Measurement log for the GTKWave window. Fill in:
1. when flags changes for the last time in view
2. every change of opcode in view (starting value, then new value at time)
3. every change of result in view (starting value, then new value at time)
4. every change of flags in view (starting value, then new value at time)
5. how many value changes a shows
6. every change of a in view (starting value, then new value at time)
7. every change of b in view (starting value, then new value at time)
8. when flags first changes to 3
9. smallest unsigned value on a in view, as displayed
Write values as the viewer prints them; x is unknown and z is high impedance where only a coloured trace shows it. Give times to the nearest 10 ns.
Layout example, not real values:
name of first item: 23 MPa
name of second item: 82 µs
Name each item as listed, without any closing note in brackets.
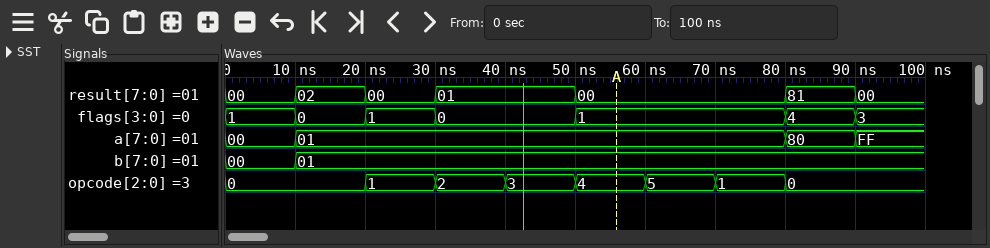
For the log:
when flags changes for the last time in view: 90 ns
every change of opcode in view: 0, 1 at 20 ns, 2 at 30 ns, 3 at 40 ns, 4 at 50 ns, 5 at 60 ns, 1 at 70 ns, 0 at 80 ns
every change of result in view: 00, 02 at 10 ns, 00 at 20 ns, 01 at 30 ns, 00 at 50 ns, 81 at 80 ns, 00 at 90 ns
every change of flags in view: 1, 0 at 10 ns, 1 at 20 ns, 0 at 30 ns, 1 at 50 ns, 4 at 80 ns, 3 at 90 ns
how many value changes a shows: 3
every change of a in view: 00, 01 at 10 ns, 80 at 80 ns, FF at 90 ns
every change of b in view: 00, 01 at 10 ns
when flags first changes to 3: 90 ns
smallest unsigned value on a in view, as displayed: 00
